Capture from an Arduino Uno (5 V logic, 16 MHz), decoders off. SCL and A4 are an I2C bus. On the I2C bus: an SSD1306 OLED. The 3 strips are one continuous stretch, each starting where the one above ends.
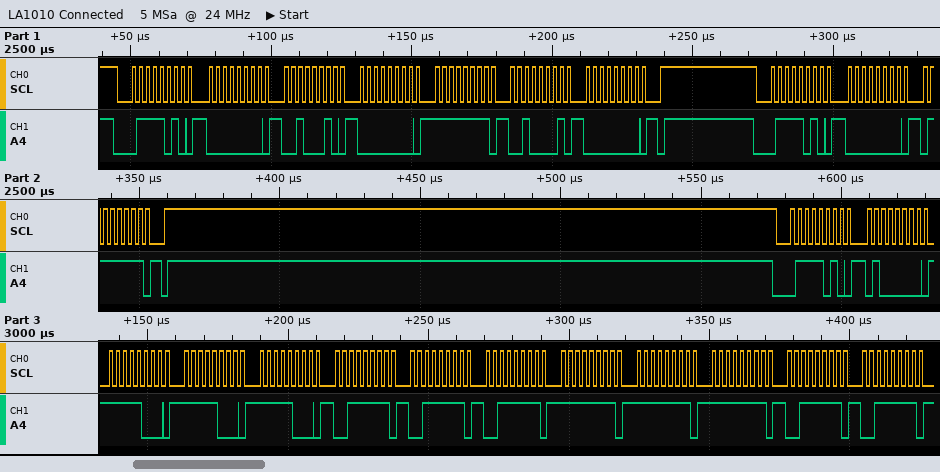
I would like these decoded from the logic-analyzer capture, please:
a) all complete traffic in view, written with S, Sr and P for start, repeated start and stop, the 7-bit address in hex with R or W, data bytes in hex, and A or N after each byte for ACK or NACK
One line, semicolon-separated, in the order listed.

S 3DW A 00 A 22 A 00 A FF A 21 A 00 A P S 3DW A 00 A 7F A P S 3DW A 40 A F8 A F8 A F8 A 3F A 3F A 3F A FF A FF A FF A 3F A 3F A
